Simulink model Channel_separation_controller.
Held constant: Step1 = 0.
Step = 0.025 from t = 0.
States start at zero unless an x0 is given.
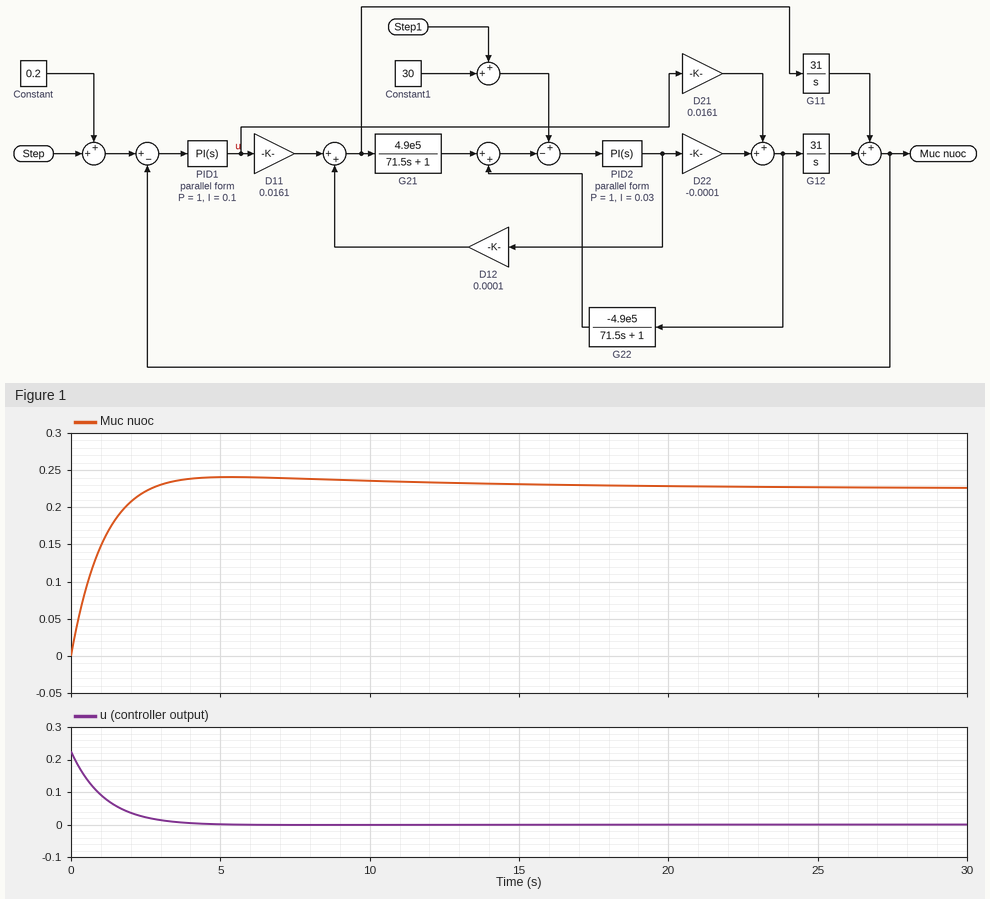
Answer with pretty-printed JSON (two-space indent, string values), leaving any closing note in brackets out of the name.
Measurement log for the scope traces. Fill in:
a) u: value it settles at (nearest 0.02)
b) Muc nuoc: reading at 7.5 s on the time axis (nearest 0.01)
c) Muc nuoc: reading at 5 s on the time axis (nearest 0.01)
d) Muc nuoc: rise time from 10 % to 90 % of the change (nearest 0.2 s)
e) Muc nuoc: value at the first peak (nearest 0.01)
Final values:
{
  "u: value it settles at": "0.00",
  "Muc nuoc: reading at 7.5 s on the time axis": "0.24",
  "Muc nuoc: reading at 5 s on the time axis": "0.24",
  "Muc nuoc: rise time from 10 % to 90 % of the change": "1.8 s",
  "Muc nuoc: value at the first peak": "0.24"
}
